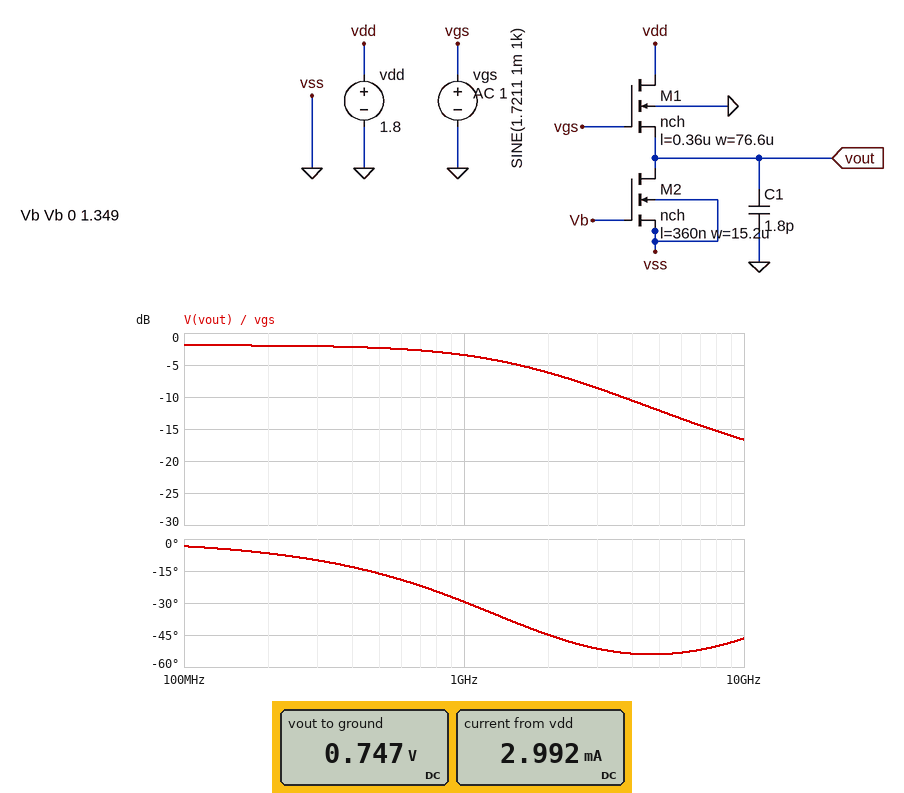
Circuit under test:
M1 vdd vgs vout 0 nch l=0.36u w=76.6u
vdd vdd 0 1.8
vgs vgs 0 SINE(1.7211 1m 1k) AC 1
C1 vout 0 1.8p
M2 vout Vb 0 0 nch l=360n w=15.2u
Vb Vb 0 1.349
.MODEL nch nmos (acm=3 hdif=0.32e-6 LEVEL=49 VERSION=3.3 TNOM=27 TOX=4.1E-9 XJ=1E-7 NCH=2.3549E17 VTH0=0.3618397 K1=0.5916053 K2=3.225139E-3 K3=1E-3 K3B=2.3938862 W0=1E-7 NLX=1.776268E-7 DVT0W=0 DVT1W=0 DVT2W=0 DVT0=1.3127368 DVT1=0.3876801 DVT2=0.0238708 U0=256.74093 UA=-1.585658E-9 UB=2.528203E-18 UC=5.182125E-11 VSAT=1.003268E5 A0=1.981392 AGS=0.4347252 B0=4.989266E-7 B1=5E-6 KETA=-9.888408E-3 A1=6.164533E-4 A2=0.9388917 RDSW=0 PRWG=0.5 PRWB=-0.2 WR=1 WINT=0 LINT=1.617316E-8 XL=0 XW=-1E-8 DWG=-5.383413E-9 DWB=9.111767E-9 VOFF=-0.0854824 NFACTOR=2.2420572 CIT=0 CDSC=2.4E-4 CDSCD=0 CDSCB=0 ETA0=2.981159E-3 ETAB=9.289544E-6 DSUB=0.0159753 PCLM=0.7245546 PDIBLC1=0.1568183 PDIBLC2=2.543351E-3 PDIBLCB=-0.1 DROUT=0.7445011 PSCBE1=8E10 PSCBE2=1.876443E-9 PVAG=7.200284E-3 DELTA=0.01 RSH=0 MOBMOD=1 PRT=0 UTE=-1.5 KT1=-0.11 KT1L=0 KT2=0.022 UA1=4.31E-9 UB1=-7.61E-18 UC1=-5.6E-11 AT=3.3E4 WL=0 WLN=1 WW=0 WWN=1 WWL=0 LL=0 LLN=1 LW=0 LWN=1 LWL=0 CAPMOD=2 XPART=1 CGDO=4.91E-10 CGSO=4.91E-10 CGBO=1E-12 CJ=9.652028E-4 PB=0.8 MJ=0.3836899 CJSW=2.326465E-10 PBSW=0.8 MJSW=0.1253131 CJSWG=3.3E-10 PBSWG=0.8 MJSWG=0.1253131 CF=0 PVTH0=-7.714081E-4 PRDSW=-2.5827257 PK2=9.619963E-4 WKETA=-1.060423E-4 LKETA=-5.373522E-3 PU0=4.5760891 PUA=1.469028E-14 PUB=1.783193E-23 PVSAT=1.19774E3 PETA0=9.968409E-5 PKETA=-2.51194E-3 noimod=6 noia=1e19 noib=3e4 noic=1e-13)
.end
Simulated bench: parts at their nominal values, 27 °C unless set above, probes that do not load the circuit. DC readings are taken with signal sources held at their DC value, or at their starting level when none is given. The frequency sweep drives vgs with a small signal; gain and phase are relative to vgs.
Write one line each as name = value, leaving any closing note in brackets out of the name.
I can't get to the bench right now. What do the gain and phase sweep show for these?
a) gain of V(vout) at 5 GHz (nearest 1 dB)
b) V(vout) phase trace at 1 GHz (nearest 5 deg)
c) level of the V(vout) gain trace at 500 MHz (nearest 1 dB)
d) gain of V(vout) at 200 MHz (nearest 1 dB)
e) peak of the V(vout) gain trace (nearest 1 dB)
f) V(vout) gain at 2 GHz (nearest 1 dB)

gain of V(vout) at 5 GHz = -12 dB
V(vout) phase trace at 1 GHz = -30 deg
level of the V(vout) gain trace at 500 MHz = -2 dB
gain of V(vout) at 200 MHz = -2 dB
peak of the V(vout) gain trace = -2 dB
V(vout) gain at 2 GHz = -6 dB
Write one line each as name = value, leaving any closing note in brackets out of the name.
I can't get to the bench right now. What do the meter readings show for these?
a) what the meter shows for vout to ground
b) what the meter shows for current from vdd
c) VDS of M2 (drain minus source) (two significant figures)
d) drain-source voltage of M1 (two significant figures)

what the meter shows for vout to ground = 0.747 V
what the meter shows for current from vdd = 2.992 mA
VDS of M2 (drain minus source) = 750 mV
drain-source voltage of M1 = 1.1 V
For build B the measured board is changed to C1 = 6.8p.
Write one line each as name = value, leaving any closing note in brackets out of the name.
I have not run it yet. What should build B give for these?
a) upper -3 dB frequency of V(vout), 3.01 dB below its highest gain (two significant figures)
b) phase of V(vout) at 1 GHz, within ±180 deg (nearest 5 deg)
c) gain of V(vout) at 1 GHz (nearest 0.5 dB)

upper -3 dB frequency of V(vout), 3.01 dB below its highest gain = 450 MHz
phase of V(vout) at 1 GHz, within ±180 deg = -60 deg
gain of V(vout) at 1 GHz = -9.5 dB
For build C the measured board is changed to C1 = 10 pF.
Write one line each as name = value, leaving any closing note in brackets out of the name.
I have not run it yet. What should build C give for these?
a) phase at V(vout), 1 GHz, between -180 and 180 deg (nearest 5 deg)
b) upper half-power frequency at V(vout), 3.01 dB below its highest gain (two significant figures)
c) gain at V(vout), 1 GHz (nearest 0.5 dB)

phase at V(vout), 1 GHz, between -180 and 180 deg = -70 deg
upper half-power frequency at V(vout), 3.01 dB below its highest gain = 310 MHz
gain at V(vout), 1 GHz = -12.5 dB
